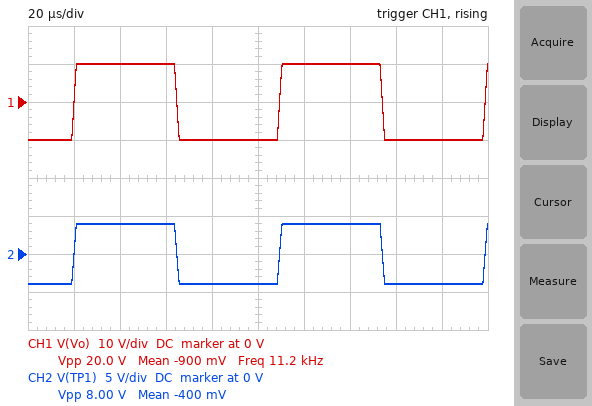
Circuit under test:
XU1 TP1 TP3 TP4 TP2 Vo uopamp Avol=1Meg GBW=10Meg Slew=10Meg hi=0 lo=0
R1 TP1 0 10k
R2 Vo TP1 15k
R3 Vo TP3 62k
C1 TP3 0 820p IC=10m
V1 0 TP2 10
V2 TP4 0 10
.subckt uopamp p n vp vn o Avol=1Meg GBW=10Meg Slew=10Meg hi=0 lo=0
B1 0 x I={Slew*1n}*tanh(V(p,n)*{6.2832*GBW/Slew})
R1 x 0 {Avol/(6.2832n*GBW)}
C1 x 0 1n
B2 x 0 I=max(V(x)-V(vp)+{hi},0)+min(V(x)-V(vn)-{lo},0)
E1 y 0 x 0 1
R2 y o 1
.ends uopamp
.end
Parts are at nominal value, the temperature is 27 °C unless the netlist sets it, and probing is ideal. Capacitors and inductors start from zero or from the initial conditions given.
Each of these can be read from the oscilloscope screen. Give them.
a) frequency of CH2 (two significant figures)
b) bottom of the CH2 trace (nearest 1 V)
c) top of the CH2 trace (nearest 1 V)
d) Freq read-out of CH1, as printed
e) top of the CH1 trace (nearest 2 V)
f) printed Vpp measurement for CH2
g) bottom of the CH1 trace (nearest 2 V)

11 kHz
-4 V
4 V
11.2 kHz
10 V
8.00 V
-10 V
